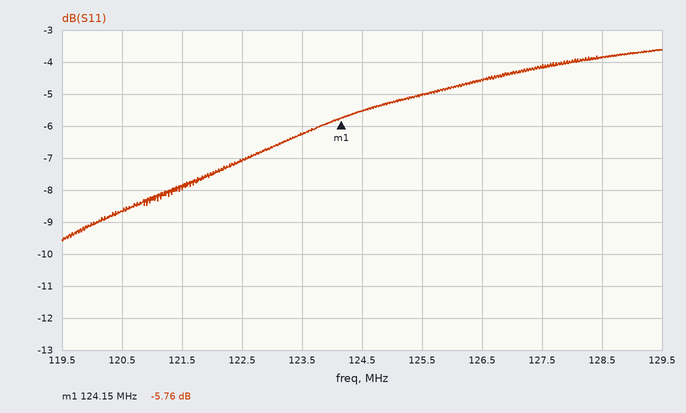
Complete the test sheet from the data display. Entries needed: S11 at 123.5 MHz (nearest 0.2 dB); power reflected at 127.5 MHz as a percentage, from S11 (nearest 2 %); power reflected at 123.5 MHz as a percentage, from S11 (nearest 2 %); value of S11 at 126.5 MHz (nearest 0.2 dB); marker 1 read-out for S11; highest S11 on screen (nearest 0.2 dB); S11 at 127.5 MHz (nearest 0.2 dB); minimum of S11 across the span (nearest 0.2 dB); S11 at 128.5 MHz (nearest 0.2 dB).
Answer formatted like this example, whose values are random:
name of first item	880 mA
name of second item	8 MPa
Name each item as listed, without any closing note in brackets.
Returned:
S11 at 123.5 MHz	-6.2 dB
power reflected at 127.5 MHz as a percentage, from S11	38 %
power reflected at 123.5 MHz as a percentage, from S11	24 %
value of S11 at 126.5 MHz	-4.6 dB
marker 1 read-out for S11	-5.76 dB
highest S11 on screen	-3.6 dB
S11 at 127.5 MHz	-4.2 dB
minimum of S11 across the span	-9.6 dB
S11 at 128.5 MHz	-3.8 dB
